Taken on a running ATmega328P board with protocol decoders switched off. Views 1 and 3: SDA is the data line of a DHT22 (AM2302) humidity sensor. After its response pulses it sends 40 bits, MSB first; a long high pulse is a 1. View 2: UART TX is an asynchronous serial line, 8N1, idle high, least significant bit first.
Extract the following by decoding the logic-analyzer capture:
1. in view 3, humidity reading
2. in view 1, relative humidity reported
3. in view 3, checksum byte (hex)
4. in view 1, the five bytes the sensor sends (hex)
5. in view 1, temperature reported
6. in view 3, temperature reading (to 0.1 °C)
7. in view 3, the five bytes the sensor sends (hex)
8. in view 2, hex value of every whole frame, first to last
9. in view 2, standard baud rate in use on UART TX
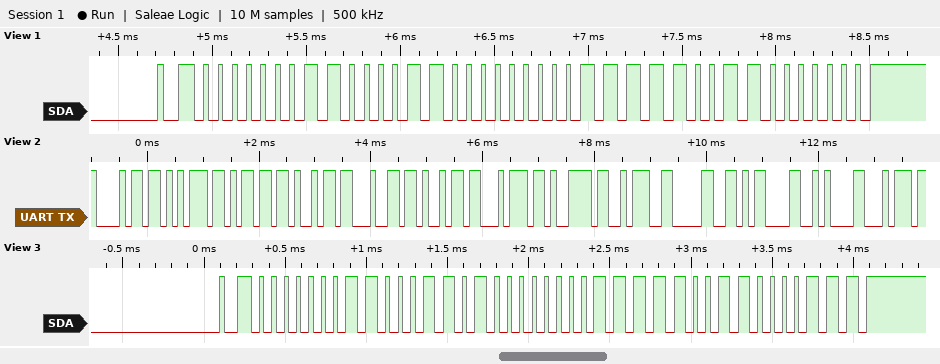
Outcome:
39.7 %
39.0 %
0x87
01 86 00 F9 80
24.9 °C
24.9 °C
01 8D 00 F9 87
68 75 6D 69 64 69 74 79 3A 30 0D 0A 74
9600 baud
